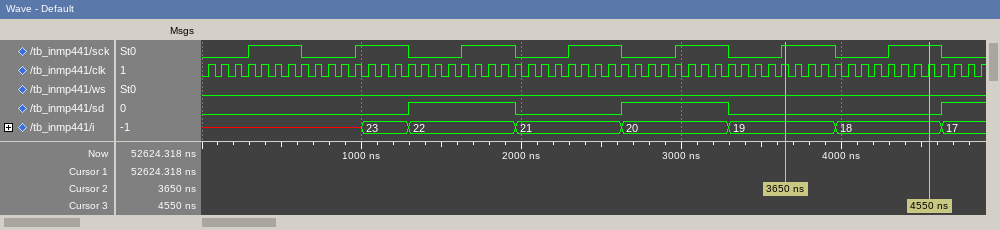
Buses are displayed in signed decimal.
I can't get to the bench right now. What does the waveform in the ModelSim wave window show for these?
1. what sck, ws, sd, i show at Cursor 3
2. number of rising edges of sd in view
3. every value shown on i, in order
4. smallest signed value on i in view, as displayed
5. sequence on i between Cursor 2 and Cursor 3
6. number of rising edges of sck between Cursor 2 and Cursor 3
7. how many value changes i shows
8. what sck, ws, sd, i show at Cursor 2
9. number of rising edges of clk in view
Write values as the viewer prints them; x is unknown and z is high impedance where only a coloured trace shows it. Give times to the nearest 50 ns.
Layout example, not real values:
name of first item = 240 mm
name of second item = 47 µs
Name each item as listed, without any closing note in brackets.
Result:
what sck, ws, sd, i show at Cursor 3 = sck=1, ws=0, sd=0, i=18
number of rising edges of sd in view = 3
every value shown on i, in order = x, 23, 22, 21, 20, 19, 18, 17
smallest signed value on i in view, as displayed = 17
sequence on i between Cursor 2 and Cursor 3 = 19, 18
number of rising edges of sck between Cursor 2 and Cursor 3 = 1
how many value changes i shows = 7
what sck, ws, sd, i show at Cursor 2 = sck=1, ws=0, sd=0, i=19
number of rising edges of clk in view = 59
